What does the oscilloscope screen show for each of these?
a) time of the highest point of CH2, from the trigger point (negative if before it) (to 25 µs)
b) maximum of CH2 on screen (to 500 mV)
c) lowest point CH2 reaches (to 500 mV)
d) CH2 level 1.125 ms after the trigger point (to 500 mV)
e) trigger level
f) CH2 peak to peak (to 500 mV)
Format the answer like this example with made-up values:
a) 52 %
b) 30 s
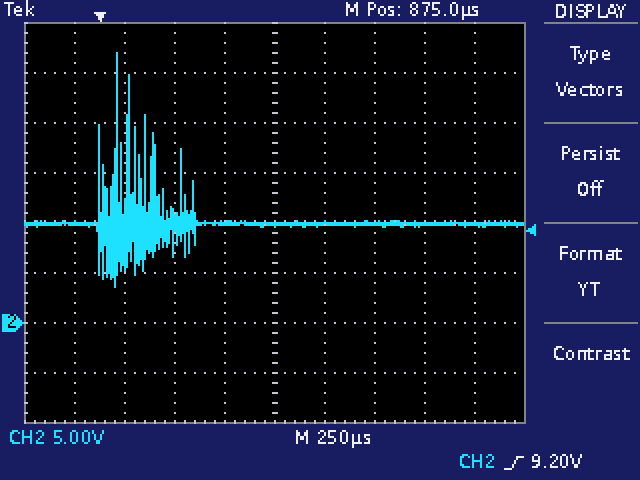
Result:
a) +100 µs
b) 27.0 V
c) 3.5 V
d) 10.0 V
e) 9.20 V
f) 23.5 V
